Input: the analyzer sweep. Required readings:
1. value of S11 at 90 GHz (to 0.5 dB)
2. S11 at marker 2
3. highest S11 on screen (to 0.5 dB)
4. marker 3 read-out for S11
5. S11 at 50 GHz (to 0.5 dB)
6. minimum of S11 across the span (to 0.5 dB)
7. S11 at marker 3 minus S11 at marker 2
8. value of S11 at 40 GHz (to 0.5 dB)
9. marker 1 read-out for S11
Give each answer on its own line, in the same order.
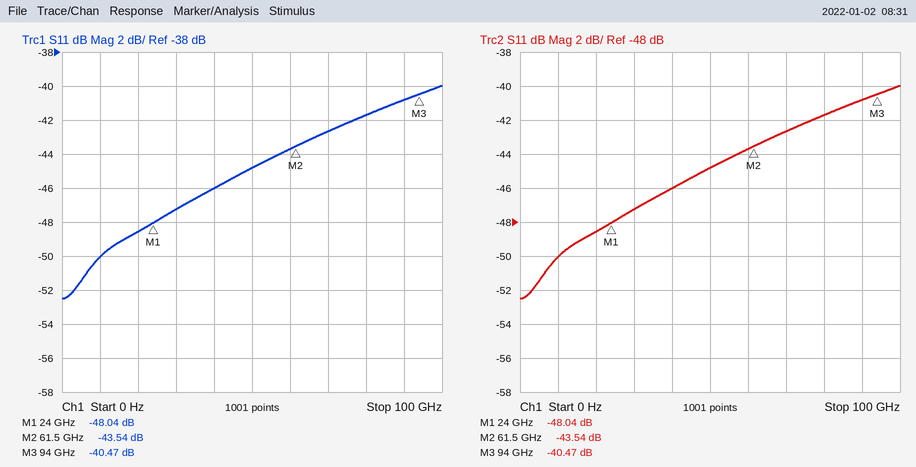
-41.0 dB
-43.54 dB
-40.0 dB
-40.47 dB
-45.0 dB
-52.5 dB
3.07 dB
-46.0 dB
-48.04 dB
